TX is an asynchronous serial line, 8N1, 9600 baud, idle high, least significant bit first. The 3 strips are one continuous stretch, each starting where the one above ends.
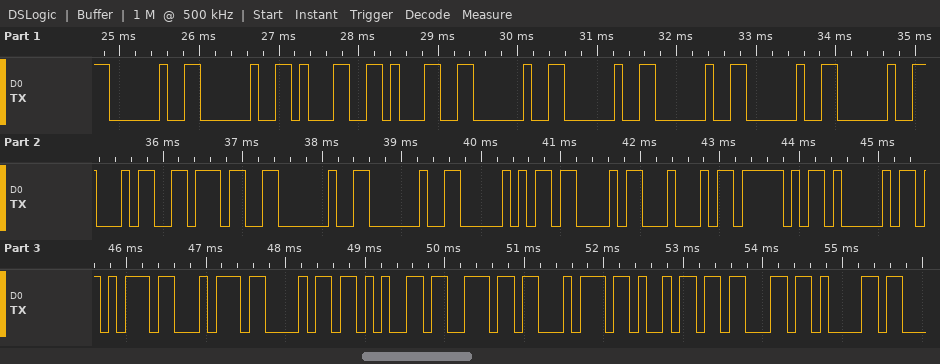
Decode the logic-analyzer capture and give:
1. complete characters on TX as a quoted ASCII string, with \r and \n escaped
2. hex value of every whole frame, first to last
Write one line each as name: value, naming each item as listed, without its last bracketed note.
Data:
complete characters on TX as a quoted ASCII string, with \r and \n escaped: "  11     47  PCD_Authentica"
hex value of every whole frame, first to last: 0x20 0x20 0x31 0x31 0x20 0x20 0x20 0x20 0x20 0x34 0x37 0x20 0x20 0x50 0x43 0x44 0x5F 0x41 0x75 0x74 0x68 0x65 0x6E 0x74 0x69 0x63 0x61
